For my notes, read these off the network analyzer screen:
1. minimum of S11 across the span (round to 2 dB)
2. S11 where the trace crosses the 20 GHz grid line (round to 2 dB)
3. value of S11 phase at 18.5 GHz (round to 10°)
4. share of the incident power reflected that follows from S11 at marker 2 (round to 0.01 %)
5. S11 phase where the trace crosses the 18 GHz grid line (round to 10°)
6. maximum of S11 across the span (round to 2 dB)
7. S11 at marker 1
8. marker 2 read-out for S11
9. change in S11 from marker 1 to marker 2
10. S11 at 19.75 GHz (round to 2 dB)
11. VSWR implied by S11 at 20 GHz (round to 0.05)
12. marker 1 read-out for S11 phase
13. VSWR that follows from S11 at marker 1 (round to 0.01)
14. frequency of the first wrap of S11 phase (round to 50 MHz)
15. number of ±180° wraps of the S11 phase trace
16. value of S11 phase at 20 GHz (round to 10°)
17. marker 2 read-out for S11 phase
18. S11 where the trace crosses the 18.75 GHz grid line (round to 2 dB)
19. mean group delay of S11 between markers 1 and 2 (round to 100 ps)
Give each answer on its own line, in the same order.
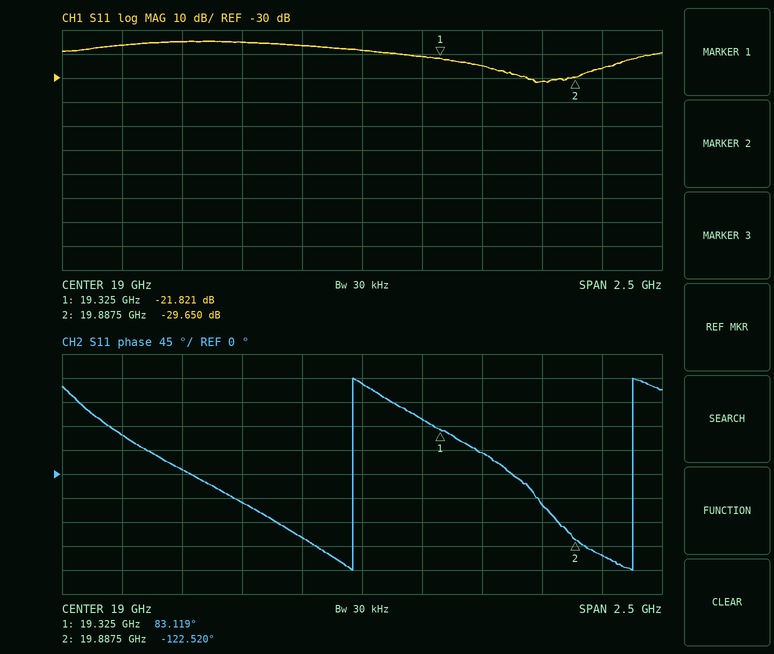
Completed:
-32 dB
-26 dB
-50°
0.11 %
70°
-14 dB
-21.821 dB
-29.650 dB
-7.829 dB
-32 dB
1.10
83.119°
1.18
18.95 GHz
2
-150°
-122.520°
-16 dB
1.0 ns
